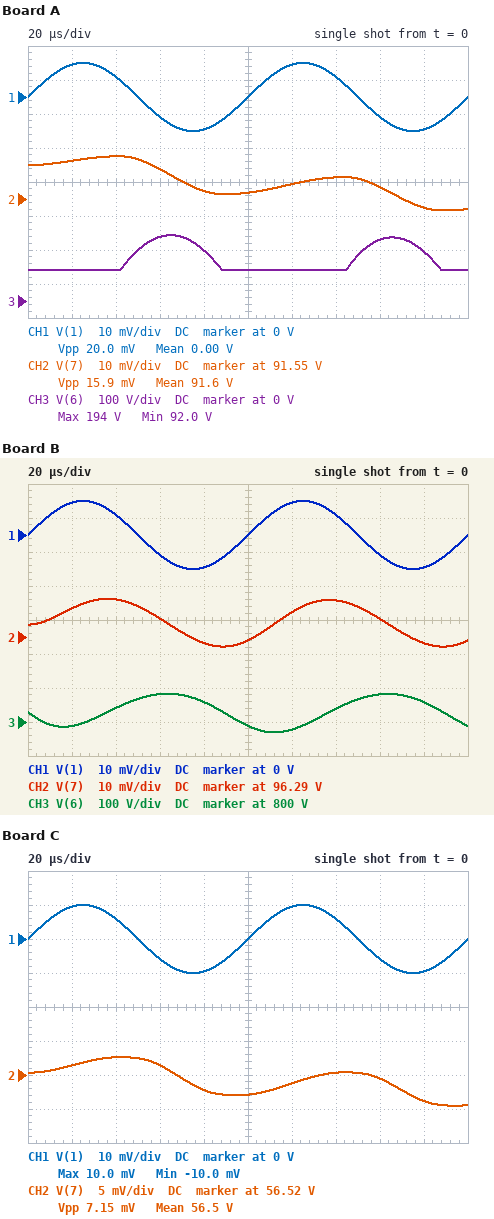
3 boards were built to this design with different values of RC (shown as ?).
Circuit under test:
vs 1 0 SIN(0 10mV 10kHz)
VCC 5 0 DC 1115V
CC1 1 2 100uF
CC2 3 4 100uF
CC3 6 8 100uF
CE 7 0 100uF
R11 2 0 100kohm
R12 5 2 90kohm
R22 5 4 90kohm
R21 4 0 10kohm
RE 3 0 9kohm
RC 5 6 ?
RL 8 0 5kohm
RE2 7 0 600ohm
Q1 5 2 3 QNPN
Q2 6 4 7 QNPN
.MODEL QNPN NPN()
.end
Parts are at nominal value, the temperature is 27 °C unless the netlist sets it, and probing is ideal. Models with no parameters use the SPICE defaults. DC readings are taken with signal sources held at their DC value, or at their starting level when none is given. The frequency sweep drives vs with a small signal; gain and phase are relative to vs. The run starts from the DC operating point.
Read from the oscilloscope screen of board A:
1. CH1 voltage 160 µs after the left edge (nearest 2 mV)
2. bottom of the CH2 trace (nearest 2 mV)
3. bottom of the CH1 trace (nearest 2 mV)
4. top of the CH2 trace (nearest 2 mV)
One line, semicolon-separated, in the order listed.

-6 mV; 91.546 V; -10 mV; 91.562 V
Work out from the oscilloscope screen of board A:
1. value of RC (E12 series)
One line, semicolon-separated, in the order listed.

6.8 kΩ
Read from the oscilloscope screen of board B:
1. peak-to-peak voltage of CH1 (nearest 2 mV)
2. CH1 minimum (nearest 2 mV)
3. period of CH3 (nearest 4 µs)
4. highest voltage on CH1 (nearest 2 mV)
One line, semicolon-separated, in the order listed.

20 mV; -10 mV; 100 µs; 10 mV
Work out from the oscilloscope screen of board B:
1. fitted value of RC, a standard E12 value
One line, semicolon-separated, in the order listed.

1.8 kΩ
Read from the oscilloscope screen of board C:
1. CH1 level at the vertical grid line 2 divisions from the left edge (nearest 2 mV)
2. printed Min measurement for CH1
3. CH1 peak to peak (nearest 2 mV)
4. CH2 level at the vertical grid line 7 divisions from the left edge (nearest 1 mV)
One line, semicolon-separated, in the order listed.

6 mV; -10.0 mV; 20 mV; 56.525 V
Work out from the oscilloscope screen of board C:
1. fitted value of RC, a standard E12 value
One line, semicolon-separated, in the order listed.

12 kΩ
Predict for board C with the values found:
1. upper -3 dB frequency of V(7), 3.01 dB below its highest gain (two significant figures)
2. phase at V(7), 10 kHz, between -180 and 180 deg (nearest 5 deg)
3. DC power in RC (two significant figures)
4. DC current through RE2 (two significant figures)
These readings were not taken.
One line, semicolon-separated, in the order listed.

3.4 kHz; -70 deg; 93 W; 94 mA
